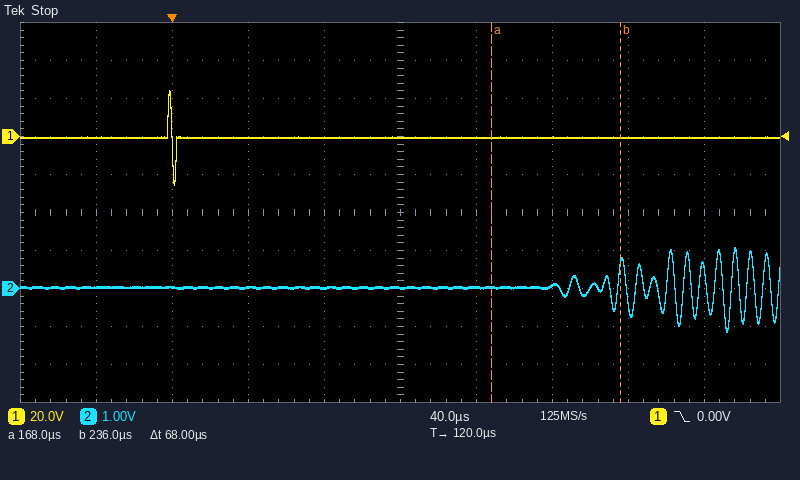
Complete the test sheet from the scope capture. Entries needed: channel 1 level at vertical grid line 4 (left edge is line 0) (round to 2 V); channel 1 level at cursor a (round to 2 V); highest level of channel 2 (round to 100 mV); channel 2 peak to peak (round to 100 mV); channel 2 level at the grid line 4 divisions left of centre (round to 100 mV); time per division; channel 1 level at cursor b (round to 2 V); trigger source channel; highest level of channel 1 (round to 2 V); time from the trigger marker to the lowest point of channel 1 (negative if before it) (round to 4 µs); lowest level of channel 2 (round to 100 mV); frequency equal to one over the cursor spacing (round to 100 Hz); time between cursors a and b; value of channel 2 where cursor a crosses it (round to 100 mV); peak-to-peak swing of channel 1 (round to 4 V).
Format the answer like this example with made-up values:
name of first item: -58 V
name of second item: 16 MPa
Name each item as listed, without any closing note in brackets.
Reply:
channel 1 level at vertical grid line 4 (left edge is line 0): 0 V
channel 1 level at cursor a: 0 V
highest level of channel 2: 1.1 V
channel 2 peak to peak: 2.2 V
channel 2 level at the grid line 4 divisions left of centre: 0.0 V
time per division: 40 µs
channel 1 level at cursor b: 0 V
trigger source channel: channel 1
highest level of channel 1: 24 V
time from the trigger marker to the lowest point of channel 1 (negative if before it): 0 µs
lowest level of channel 2: -1.1 V
frequency equal to one over the cursor spacing: 14.7 kHz
time between cursors a and b: 68 µs
value of channel 2 where cursor a crosses it: 0.0 V
peak-to-peak swing of channel 1: 48 V
